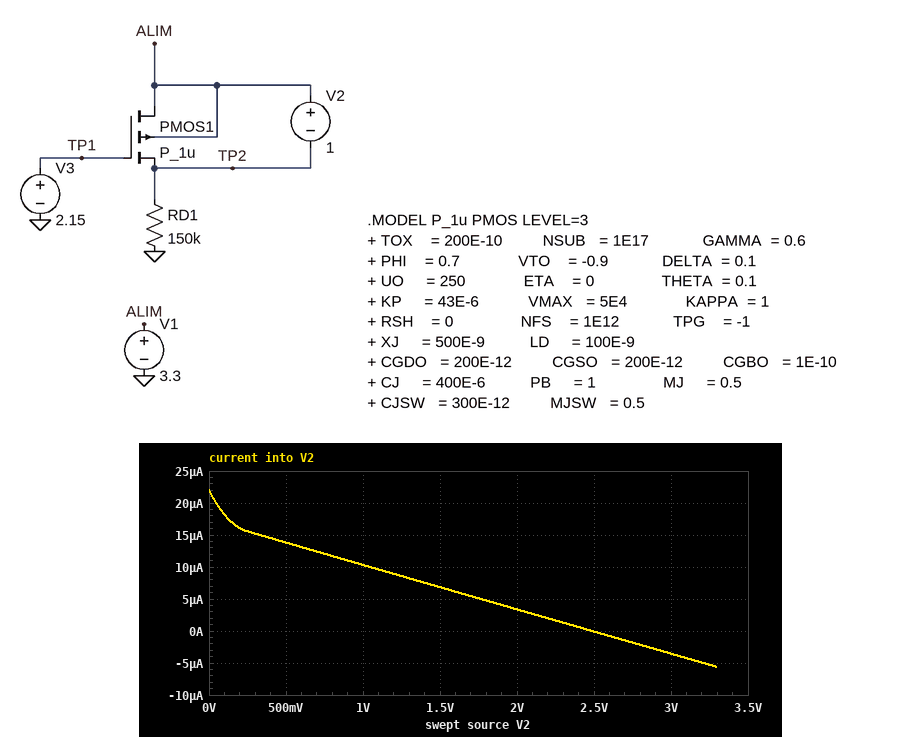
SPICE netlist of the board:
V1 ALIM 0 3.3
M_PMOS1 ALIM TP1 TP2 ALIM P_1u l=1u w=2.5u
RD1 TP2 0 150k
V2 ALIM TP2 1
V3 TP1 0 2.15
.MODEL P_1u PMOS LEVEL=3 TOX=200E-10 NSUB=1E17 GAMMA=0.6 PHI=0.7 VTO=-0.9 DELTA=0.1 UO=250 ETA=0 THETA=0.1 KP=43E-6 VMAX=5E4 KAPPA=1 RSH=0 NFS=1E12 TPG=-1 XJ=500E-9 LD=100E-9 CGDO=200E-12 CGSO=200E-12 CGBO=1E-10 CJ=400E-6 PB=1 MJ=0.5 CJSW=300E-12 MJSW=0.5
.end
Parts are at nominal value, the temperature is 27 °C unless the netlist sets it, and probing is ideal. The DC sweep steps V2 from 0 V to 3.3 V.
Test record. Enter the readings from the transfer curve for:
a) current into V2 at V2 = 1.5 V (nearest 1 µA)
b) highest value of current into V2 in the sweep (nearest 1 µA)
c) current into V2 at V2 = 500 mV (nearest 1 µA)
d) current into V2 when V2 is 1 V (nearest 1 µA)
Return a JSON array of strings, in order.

["7 µA", "22 µA", "14 µA", "10 µA"]
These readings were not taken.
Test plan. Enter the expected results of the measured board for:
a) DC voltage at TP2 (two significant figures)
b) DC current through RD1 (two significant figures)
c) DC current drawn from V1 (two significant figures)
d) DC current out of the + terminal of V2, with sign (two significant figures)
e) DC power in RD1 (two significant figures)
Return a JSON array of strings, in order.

["2.3 V", "15 µA", "15 µA", "-10 µA", "35 µW"]
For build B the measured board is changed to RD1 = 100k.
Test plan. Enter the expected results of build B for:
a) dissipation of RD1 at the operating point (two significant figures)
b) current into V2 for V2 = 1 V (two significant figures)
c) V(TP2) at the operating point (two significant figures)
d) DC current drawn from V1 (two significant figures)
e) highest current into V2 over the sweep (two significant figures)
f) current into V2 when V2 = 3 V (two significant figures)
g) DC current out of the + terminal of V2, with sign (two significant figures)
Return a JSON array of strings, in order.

["53 µW", "18 µA", "2.3 V", "23 µA", "33 µA", "-2.5 µA", "-18 µA"]
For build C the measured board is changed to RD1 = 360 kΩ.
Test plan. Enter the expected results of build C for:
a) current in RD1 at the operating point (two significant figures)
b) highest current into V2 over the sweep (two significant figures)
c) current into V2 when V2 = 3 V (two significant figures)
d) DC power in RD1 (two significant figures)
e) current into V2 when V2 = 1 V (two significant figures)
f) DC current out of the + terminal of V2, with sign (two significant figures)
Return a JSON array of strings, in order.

["6.4 µA", "9.2 µA", "-4.7 µA", "15 µW", "1.4 µA", "-1.4 µA"]
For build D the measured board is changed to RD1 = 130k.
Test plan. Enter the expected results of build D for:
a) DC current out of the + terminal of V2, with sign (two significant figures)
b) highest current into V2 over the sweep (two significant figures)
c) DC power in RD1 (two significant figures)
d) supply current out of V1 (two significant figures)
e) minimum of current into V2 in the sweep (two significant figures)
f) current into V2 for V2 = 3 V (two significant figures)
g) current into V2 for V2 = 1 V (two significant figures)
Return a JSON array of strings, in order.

["-13 µA", "25 µA", "41 µW", "18 µA", "-5.6 µA", "-3.2 µA", "13 µA"]
